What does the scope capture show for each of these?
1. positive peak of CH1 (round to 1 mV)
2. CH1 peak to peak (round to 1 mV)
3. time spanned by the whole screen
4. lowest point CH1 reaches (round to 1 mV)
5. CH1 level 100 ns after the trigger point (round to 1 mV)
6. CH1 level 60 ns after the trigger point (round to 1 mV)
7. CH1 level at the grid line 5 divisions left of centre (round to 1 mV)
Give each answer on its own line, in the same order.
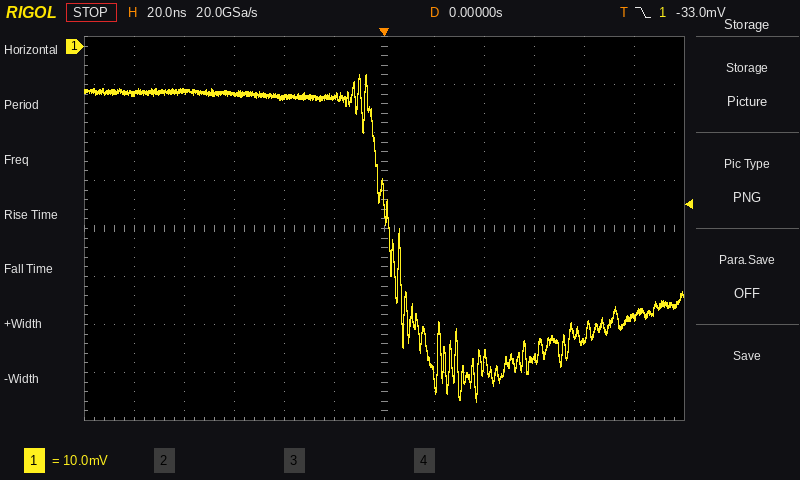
-6 mV
68 mV
240 ns
-74 mV
-56 mV
-65 mV
-10 mV
